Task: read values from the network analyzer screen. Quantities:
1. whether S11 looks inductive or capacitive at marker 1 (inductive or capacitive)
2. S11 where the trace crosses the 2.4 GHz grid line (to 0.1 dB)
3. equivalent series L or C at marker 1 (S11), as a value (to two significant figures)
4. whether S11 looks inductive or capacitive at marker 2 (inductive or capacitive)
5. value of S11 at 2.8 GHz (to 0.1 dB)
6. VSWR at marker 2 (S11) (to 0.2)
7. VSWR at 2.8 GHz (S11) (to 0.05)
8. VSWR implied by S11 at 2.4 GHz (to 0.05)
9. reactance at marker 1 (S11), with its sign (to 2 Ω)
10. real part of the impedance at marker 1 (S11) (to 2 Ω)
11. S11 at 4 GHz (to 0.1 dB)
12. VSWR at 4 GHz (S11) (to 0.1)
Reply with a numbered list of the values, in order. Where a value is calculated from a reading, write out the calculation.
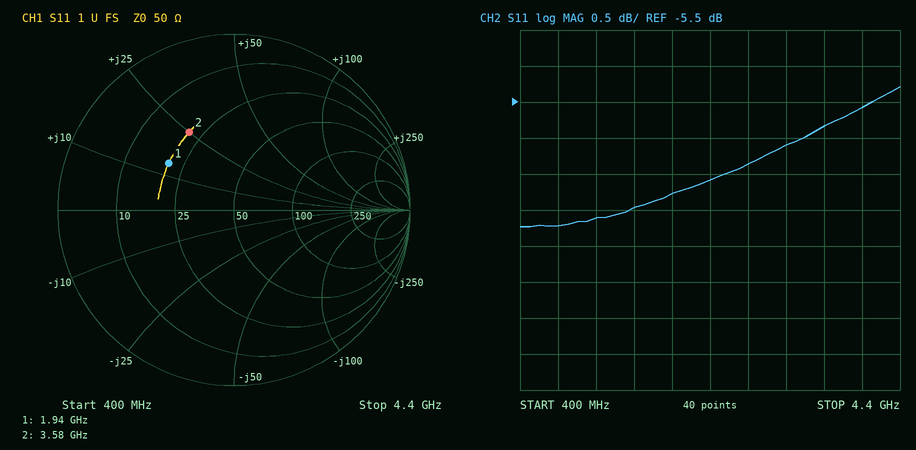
1. inductive
2. -6.6 dB
3. L = 14 Ω/(2π × 1.94 GHz) ≈ 1.1 nH
4. inductive
5. -6.4 dB
6. 3.0
7. |Γ| = 10^(-6.4/20) = 0.4786; VSWR = (1 + 0.4786)/(1 − 0.4786) ≈ 2.84, so 2.85 to the nearest 0.05
8. |Γ| = 10^(-6.6/20) = 0.4677; VSWR = (1 + 0.4677)/(1 − 0.4677) ≈ 2.76, so 2.75 to the nearest 0.05
9. +14 Ω
10. 20 Ω
11. -5.6 dB
12. |Γ| = 10^(-5.6/20) = 0.5248; VSWR = (1 + 0.5248)/(1 − 0.5248) ≈ 3.2
